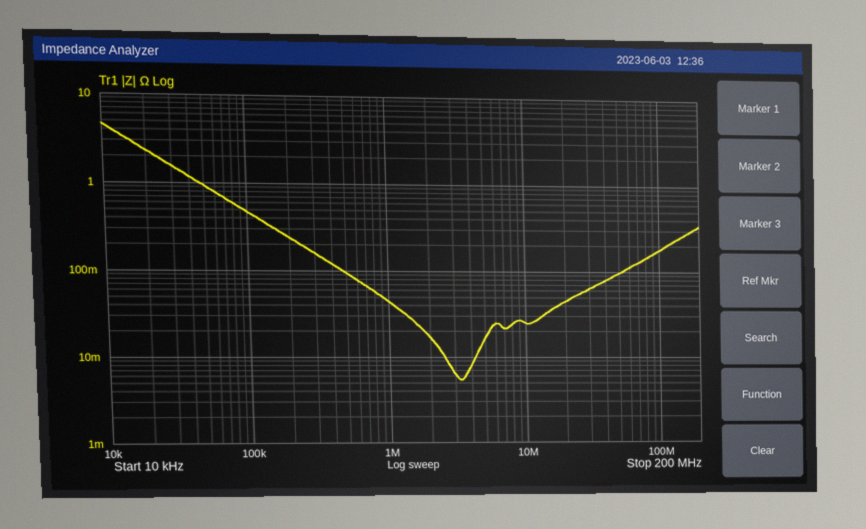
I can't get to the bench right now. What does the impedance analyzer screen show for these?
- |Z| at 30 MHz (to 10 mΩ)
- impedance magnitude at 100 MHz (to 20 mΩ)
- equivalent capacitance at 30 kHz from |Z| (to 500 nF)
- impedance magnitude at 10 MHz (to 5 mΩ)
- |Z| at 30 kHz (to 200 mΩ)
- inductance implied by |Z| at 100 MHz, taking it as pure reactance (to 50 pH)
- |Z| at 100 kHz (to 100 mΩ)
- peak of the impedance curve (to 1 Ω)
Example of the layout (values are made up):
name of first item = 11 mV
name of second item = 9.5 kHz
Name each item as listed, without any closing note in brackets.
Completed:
|Z| at 30 MHz = 60 mΩ
impedance magnitude at 100 MHz = 180 mΩ
equivalent capacitance at 30 kHz from |Z| = 3.5 µF
impedance magnitude at 10 MHz = 25 mΩ
|Z| at 30 kHz = 1.6 Ω
inductance implied by |Z| at 100 MHz, taking it as pure reactance = 300 pH
|Z| at 100 kHz = 500 mΩ
peak of the impedance curve = 5 Ω
